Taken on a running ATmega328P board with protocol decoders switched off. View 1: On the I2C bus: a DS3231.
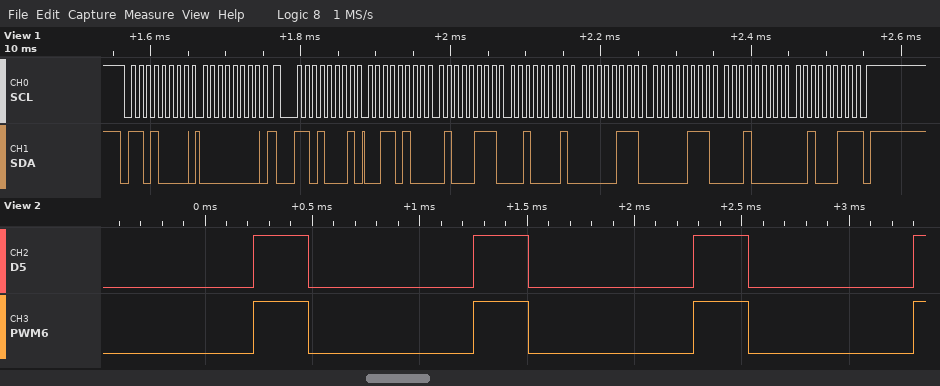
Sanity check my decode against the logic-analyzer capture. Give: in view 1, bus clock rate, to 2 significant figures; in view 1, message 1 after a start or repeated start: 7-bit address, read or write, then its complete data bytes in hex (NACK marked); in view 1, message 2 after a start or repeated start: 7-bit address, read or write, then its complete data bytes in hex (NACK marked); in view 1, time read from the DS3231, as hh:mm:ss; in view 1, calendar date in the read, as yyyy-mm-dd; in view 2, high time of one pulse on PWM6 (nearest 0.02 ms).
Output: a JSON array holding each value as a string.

["100 kHz", "0x68 write: 00", "0x68 read: 34 47 21 07 07 10 23 NACK", "21:47:34", "2023-10-07", "0.26 ms"]
